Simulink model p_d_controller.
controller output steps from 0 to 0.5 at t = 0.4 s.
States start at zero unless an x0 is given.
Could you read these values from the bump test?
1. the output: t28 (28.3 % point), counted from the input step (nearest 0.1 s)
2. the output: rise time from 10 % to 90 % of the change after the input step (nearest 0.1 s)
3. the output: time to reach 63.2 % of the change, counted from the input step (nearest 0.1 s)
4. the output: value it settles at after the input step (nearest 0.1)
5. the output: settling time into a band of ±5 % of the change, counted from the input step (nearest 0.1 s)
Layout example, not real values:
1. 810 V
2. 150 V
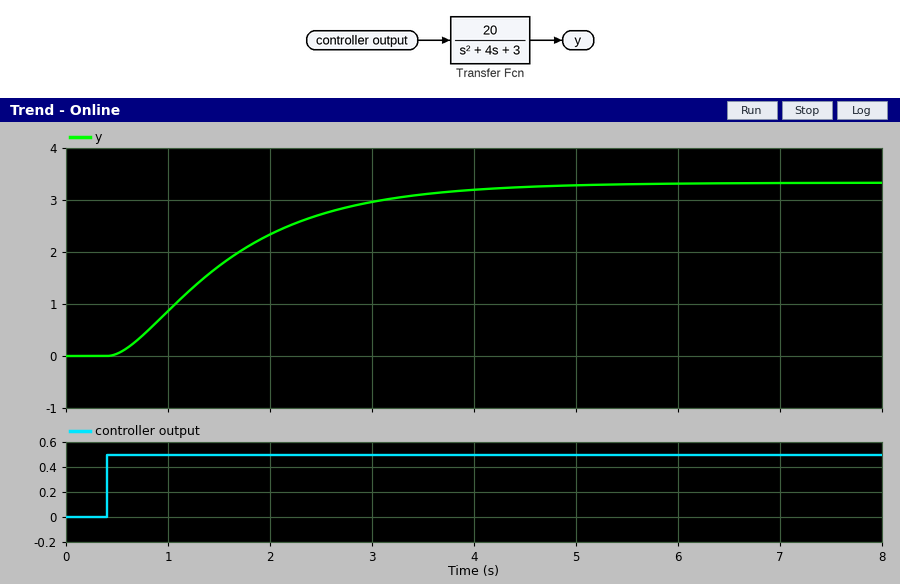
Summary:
1. 0.6 s
2. 2.4 s
3. 1.4 s
4. 3.3
5. 3.4 s
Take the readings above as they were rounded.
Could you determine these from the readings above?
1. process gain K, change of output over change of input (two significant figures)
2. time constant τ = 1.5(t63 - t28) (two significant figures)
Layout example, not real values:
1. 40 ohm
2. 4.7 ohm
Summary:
1. 6.6
2. 1.2 s
